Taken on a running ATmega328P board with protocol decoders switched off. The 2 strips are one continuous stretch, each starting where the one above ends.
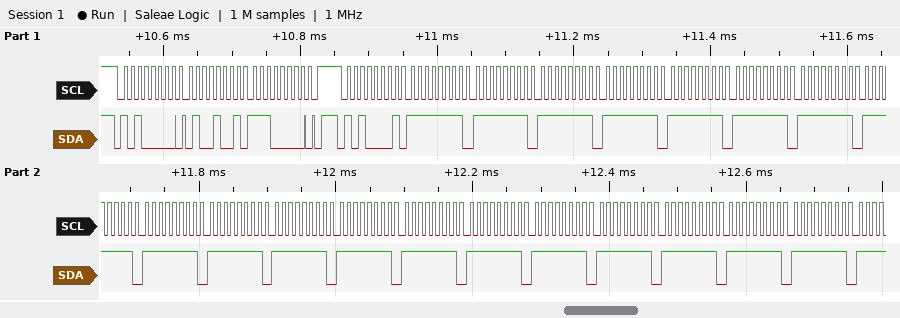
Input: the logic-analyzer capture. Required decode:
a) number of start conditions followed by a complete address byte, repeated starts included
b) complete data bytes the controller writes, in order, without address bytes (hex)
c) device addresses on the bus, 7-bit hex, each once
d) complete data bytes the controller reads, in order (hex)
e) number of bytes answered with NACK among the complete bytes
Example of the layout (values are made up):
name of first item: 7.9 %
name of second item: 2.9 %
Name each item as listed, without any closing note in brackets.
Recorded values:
number of start conditions followed by a complete address byte, repeated starts included: 2
complete data bytes the controller writes, in order, without address bytes: 49 E0
device addresses on the bus, 7-bit hex, each once: 0x50
complete data bytes the controller reads, in order: FF FF FF FF FF FF FF FF FF FF FF FF FF FF FF FF FF FF FF
number of bytes answered with NACK among the complete bytes: 0
